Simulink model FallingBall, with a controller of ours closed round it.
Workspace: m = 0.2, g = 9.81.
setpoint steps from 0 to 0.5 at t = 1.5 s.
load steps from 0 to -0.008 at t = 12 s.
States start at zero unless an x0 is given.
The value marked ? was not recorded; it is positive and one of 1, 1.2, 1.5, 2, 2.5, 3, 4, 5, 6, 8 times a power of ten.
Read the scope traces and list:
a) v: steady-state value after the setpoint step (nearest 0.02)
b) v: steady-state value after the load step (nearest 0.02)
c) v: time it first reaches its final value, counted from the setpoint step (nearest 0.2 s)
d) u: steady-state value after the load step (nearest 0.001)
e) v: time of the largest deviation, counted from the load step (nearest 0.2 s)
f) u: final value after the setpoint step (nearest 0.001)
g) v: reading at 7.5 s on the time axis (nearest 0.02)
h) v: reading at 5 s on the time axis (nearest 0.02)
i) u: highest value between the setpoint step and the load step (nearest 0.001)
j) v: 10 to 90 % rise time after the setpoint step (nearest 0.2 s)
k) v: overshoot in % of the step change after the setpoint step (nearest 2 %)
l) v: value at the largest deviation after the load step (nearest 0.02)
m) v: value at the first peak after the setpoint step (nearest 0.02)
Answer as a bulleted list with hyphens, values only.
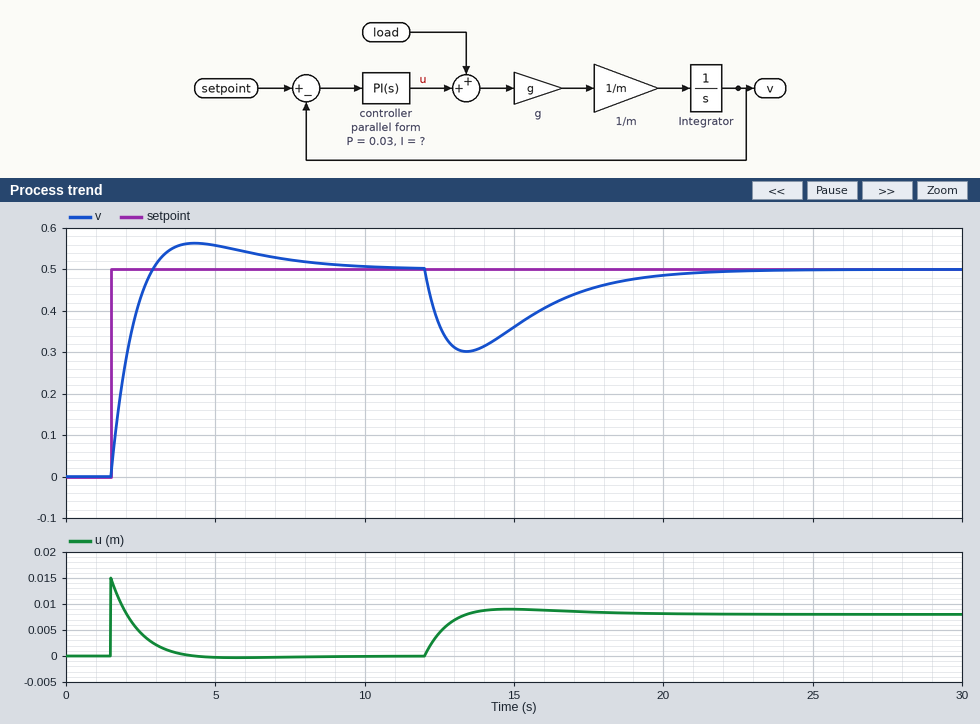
- 0.50
- 0.50
- 1.4 s
- 0.008
- 1.4 s
- 0.000
- 0.52
- 0.56
- 0.015
- 1.0 s
- 12 %
- 0.30
- 0.56
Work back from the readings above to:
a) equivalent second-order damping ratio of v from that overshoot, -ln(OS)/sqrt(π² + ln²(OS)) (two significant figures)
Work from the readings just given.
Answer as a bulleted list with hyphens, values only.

- 0.56
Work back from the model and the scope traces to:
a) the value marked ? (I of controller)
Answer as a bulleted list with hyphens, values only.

- 0.01
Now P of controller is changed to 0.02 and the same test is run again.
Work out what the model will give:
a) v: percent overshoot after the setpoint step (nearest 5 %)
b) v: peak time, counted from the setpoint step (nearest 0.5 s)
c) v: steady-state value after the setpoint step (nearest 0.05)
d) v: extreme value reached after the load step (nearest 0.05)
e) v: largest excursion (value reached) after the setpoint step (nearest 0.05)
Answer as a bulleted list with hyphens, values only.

- 20 %
- 3.0 s
- 0.50
- 0.25
- 0.60
